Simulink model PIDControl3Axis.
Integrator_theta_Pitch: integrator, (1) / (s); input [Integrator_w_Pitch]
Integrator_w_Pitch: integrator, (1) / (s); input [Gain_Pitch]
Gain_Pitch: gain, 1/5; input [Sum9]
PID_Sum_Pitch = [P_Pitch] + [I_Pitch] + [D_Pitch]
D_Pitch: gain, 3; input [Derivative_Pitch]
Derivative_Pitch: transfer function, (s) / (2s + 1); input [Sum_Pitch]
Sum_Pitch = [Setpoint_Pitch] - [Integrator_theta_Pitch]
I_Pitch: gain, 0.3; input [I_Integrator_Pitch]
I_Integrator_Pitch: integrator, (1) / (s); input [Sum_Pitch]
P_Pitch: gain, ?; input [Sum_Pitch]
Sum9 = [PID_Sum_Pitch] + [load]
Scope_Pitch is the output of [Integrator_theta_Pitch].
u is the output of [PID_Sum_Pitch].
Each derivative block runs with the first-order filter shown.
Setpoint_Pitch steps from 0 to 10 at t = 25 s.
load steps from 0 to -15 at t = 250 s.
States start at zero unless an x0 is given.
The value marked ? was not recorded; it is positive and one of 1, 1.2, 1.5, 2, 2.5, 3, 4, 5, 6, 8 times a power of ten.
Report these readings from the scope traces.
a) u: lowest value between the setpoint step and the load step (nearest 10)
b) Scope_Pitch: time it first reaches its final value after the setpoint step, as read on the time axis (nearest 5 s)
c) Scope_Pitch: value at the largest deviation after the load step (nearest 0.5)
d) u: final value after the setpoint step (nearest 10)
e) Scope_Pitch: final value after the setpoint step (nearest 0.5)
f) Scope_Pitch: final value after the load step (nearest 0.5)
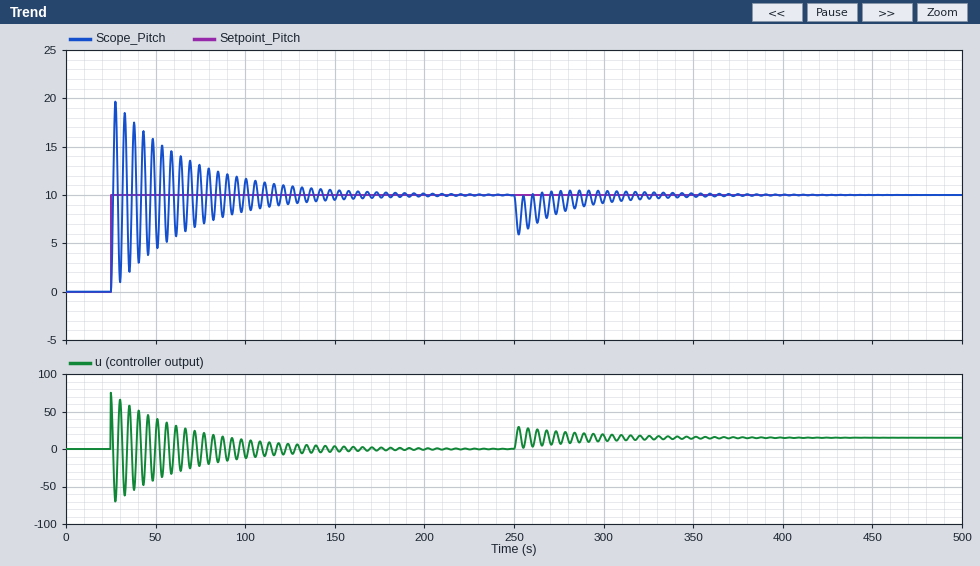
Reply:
-70
25 s
6.0
0
10.0
10.0
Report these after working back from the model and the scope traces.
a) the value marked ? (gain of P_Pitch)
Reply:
6
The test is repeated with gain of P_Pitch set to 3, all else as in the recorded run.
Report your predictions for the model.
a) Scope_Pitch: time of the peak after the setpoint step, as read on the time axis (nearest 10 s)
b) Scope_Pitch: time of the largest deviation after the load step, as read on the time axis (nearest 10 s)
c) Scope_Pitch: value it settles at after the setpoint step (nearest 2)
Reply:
30 s
250 s
10
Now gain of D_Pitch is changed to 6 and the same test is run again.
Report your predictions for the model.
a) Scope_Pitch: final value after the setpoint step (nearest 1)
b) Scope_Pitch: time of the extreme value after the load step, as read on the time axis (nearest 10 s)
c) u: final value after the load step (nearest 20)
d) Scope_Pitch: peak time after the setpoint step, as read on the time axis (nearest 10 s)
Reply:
10
250 s
20
30 s
